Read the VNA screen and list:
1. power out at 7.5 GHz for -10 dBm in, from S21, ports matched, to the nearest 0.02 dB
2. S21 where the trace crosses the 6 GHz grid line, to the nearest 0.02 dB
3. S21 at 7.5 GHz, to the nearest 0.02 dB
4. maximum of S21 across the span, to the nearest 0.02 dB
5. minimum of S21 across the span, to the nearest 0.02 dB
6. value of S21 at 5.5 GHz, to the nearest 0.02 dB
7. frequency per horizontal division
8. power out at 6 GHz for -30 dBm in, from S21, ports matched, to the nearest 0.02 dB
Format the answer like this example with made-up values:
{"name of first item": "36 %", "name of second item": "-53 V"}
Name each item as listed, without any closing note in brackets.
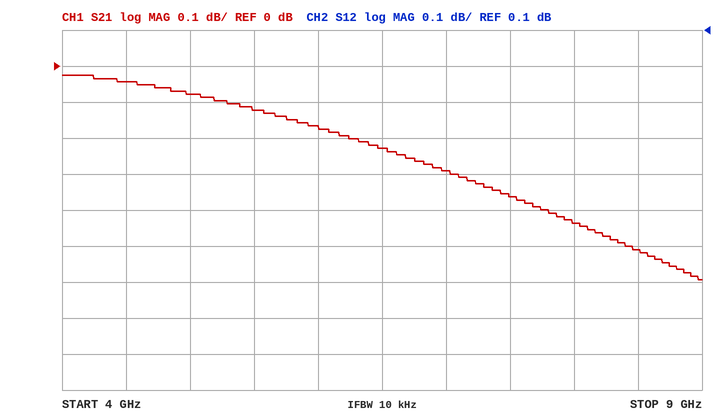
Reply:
{"power out at 7.5 GHz for -10 dBm in, from S21, ports matched, to the nearest 0.02 dB": "-10.36 dBm", "S21 where the trace crosses the 6 GHz grid line, to the nearest 0.02 dB": "-0.16 dB", "S21 at 7.5 GHz, to the nearest 0.02 dB": "-0.36 dB", "maximum of S21 across the span, to the nearest 0.02 dB": "-0.02 dB", "minimum of S21 across the span, to the nearest 0.02 dB": "-0.60 dB", "value of S21 at 5.5 GHz, to the nearest 0.02 dB": "-0.12 dB", "frequency per horizontal division": "500 MHz", "power out at 6 GHz for -30 dBm in, from S21, ports matched, to the nearest 0.02 dB": "-30.16 dBm"}
